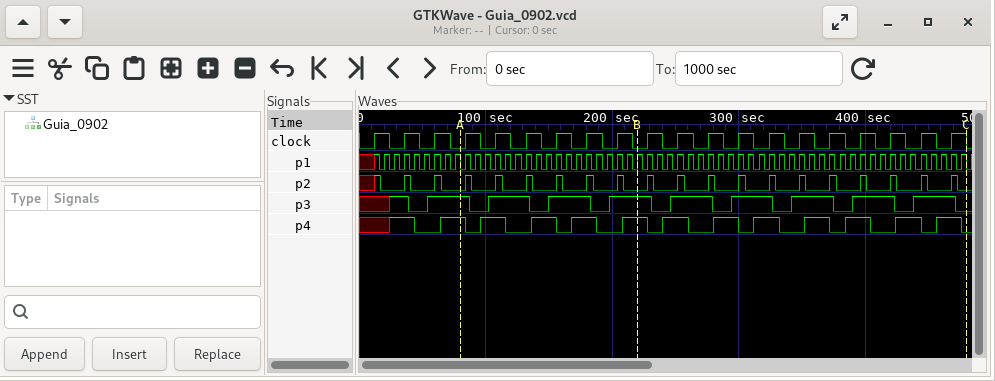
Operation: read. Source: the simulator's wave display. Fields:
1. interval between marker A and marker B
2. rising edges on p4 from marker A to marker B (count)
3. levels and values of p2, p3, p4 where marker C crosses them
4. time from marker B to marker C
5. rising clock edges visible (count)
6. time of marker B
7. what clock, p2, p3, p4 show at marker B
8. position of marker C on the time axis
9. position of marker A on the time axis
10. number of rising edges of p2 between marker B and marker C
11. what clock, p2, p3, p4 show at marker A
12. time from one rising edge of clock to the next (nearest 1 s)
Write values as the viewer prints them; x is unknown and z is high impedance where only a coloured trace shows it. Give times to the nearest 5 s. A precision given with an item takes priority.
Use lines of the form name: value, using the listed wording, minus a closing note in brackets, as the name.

interval between marker A and marker B: 140 s
rising edges on p4 from marker A to marker B: 4
levels and values of p2, p3, p4 where marker C crosses them: p2=0, p3=0, p4=0
time from marker B to marker C: 260 s
rising clock edges visible: 20
time of marker B: 220 s
what clock, p2, p3, p4 show at marker B: clock=0, p2=0, p3=1, p4=1
position of marker C on the time axis: 480 s
position of marker A on the time axis: 80 s
number of rising edges of p2 between marker B and marker C: 11
what clock, p2, p3, p4 show at marker A: clock=0, p2=0, p3=1, p4=1
time from one rising edge of clock to the next: 24 s
